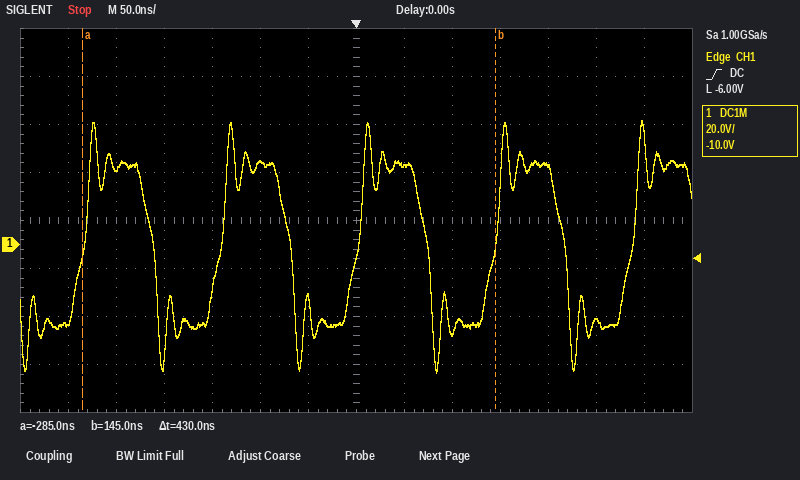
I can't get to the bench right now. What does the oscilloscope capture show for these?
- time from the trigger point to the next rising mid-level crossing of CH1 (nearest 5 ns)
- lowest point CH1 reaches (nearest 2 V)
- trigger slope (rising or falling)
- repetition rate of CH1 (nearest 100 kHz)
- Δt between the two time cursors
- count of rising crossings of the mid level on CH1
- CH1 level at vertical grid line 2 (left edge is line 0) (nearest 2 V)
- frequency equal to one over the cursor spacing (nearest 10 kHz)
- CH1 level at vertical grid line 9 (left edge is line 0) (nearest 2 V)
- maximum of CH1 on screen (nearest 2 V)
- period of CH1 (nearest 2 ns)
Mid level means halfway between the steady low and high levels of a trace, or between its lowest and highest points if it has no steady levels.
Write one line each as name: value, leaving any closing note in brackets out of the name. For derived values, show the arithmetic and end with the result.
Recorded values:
time from the trigger point to the next rising mid-level crossing of CH1: 5 ns
lowest point CH1 reaches: -54 V
trigger slope: rising
repetition rate of CH1: 1 / 142 ns ≈ 7.0 MHz
Δt between the two time cursors: 430 ns
count of rising crossings of the mid level on CH1: 5
CH1 level at vertical grid line 2 (left edge is line 0): 32 V
frequency equal to one over the cursor spacing: 1 / 430 ns ≈ 2.33 MHz
CH1 level at vertical grid line 9 (left edge is line 0): -36 V
maximum of CH1 on screen: 52 V
period of CH1: 142 ns
